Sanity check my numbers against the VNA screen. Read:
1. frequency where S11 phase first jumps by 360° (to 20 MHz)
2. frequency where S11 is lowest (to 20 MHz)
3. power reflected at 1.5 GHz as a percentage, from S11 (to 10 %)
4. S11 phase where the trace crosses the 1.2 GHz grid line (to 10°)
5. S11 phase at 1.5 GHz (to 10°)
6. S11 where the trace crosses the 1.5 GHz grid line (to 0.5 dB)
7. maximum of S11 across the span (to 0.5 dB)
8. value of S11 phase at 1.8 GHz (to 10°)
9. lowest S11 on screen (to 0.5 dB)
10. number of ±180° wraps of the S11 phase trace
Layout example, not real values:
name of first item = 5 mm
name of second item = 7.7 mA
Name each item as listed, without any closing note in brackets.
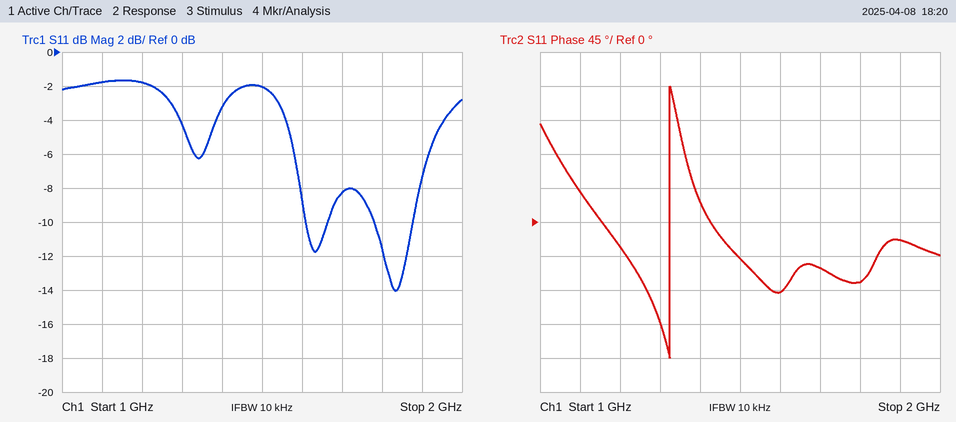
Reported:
frequency where S11 phase first jumps by 360° = 1.32 GHz
frequency where S11 is lowest = 1.84 GHz
power reflected at 1.5 GHz as a percentage, from S11 = 60 %
S11 phase where the trace crosses the 1.2 GHz grid line = -30°
S11 phase at 1.5 GHz = -50°
S11 where the trace crosses the 1.5 GHz grid line = -2.0 dB
maximum of S11 across the span = -1.5 dB
value of S11 phase at 1.8 GHz = -80°
lowest S11 on screen = -14.0 dB
number of ±180° wraps of the S11 phase trace = 1
